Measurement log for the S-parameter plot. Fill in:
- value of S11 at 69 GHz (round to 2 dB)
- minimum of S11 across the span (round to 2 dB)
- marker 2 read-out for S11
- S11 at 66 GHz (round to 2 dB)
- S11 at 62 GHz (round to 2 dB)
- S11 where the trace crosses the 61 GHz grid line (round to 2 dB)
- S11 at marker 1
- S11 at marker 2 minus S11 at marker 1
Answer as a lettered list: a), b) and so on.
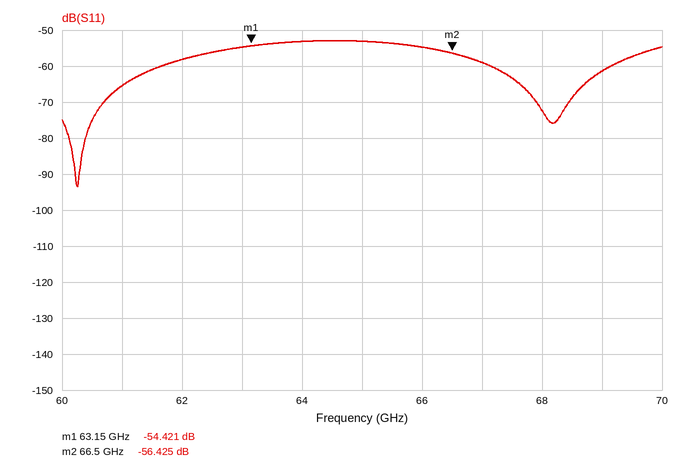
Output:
a) -62 dB
b) -94 dB
c) -56.425 dB
d) -54 dB
e) -58 dB
f) -66 dB
g) -54.421 dB
h) -2.004 dB
